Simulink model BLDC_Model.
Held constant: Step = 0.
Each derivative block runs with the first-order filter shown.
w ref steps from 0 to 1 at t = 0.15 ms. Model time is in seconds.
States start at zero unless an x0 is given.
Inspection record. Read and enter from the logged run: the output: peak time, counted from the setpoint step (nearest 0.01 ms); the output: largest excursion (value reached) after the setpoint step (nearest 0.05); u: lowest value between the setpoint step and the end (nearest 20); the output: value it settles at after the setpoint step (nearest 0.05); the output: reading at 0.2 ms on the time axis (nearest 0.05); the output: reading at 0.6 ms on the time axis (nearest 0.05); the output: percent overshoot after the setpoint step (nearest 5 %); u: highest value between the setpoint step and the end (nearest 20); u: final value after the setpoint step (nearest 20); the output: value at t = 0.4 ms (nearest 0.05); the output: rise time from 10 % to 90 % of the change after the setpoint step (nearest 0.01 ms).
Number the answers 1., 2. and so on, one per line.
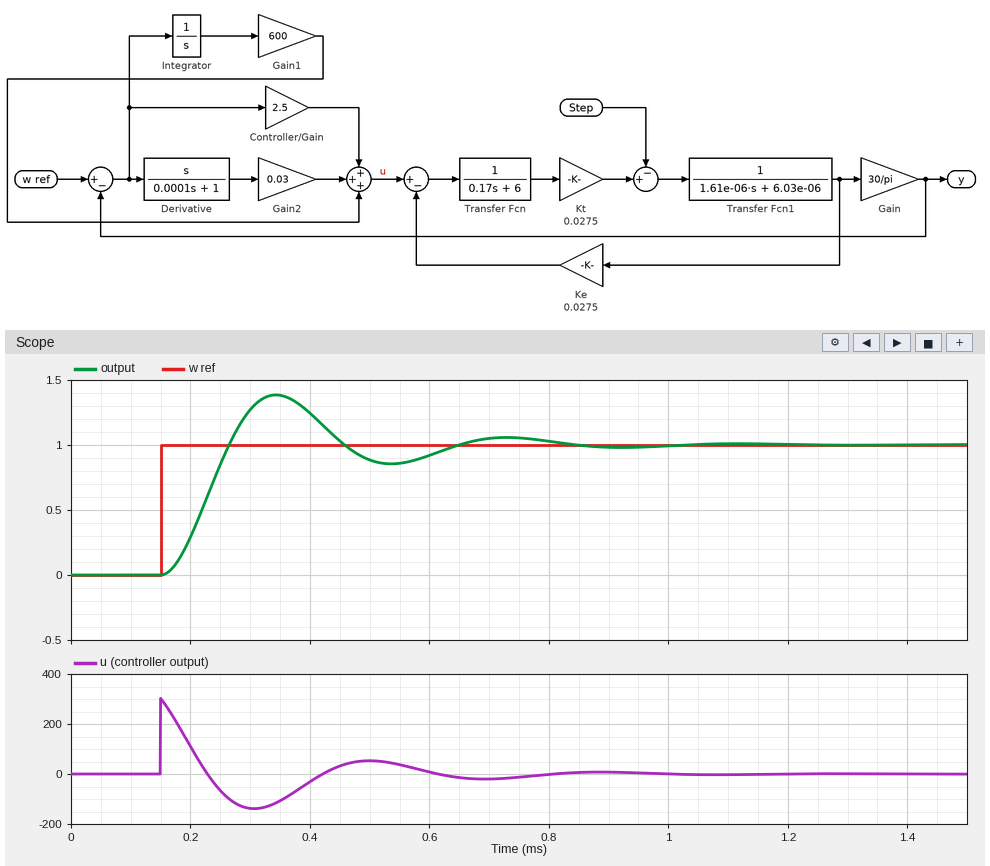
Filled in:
1. 0.19 ms
2. 1.40
3. -140
4. 1.00
5. 0.30
6. 0.90
7. 40 %
8. 300
9. 0
10. 1.25
11. 0.08 ms
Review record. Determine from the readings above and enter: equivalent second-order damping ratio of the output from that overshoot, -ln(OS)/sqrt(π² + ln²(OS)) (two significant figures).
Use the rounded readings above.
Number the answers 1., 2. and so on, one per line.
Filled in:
1. 0.28
